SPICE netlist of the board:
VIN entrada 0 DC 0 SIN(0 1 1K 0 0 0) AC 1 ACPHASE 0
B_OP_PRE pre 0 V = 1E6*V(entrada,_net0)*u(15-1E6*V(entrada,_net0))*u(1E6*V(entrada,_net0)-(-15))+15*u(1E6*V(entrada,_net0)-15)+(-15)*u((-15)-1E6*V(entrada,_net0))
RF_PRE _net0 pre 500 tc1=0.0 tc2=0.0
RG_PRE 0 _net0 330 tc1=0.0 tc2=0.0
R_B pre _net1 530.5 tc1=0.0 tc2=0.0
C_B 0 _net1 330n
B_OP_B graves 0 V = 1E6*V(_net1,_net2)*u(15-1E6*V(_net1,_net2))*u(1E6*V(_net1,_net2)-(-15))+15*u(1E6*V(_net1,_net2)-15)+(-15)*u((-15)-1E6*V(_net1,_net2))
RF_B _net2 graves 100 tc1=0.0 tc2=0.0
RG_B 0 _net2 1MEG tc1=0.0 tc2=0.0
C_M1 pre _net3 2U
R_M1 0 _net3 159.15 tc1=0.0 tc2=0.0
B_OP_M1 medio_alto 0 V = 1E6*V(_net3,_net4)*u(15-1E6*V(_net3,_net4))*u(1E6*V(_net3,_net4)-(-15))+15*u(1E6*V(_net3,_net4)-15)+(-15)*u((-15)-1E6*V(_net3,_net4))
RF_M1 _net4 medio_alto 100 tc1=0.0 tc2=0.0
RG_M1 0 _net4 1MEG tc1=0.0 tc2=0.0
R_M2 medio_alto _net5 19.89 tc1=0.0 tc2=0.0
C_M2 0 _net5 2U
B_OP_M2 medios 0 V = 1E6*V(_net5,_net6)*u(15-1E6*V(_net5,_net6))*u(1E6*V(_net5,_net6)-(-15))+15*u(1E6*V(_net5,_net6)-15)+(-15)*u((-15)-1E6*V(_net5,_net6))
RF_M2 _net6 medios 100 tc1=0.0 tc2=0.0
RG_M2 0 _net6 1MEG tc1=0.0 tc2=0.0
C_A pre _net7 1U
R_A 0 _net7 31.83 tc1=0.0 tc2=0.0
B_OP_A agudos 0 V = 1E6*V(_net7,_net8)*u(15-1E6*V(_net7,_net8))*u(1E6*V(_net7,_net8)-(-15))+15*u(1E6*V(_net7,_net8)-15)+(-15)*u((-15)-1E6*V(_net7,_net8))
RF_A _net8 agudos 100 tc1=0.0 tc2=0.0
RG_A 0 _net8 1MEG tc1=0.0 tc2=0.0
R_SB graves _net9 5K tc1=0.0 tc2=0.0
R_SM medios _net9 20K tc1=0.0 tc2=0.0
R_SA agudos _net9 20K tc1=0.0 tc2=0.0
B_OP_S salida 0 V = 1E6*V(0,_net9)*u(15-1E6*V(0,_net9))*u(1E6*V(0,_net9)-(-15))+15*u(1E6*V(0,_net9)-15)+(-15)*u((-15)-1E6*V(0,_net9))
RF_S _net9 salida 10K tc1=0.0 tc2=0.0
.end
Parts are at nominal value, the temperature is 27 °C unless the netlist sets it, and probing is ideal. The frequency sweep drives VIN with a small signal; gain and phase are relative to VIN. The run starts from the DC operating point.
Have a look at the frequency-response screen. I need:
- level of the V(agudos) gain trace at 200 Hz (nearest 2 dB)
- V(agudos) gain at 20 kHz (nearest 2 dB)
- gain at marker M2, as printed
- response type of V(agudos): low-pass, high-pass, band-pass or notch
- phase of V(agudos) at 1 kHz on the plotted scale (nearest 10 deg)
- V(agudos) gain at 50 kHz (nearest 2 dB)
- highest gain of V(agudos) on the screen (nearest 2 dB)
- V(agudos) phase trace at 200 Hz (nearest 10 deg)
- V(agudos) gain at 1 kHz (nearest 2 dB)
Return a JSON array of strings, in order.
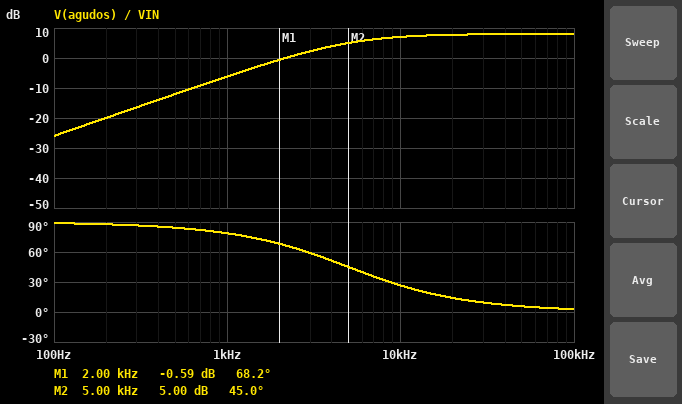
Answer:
["-20 dB", "8 dB", "5.00 dB", "high-pass", "80 deg", "8 dB", "8 dB", "90 deg", "-6 dB"]
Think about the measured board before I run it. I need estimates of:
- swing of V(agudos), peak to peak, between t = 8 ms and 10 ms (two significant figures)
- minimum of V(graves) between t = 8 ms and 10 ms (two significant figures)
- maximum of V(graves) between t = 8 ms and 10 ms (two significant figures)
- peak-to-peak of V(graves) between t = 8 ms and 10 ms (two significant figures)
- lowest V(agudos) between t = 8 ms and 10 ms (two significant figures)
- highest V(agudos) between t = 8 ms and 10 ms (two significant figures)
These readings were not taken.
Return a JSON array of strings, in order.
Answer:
["990 mV", "-1.7 V", "1.7 V", "3.4 V", "-490 mV", "490 mV"]
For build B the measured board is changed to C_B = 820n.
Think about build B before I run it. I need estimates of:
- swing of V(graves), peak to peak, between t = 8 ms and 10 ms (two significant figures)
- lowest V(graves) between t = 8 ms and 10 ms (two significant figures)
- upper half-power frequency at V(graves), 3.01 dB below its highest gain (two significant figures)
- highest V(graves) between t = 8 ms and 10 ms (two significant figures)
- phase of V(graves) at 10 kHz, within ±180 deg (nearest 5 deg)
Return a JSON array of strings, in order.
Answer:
["1.7 V", "-860 mV", "370 Hz", "860 mV", "-90 deg"]
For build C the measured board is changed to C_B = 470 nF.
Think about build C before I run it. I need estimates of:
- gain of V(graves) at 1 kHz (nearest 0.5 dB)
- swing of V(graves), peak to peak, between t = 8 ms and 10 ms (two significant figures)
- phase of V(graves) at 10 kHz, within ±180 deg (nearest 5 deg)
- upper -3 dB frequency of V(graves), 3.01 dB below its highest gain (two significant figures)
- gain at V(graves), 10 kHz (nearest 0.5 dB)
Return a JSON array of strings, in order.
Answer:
["2.5 dB", "2.7 V", "-85 deg", "640 Hz", "-16.0 dB"]
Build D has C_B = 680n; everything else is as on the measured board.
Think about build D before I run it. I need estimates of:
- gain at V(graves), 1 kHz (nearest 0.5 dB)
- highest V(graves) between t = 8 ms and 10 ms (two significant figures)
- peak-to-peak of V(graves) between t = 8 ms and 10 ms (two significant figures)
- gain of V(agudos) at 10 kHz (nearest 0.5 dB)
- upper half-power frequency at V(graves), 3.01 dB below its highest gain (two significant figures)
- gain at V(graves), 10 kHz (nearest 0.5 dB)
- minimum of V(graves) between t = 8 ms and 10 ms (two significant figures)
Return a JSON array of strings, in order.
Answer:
["0 dB", "1.0 V", "2.0 V", "7.0 dB", "440 Hz", "-19.0 dB", "-1.0 V"]
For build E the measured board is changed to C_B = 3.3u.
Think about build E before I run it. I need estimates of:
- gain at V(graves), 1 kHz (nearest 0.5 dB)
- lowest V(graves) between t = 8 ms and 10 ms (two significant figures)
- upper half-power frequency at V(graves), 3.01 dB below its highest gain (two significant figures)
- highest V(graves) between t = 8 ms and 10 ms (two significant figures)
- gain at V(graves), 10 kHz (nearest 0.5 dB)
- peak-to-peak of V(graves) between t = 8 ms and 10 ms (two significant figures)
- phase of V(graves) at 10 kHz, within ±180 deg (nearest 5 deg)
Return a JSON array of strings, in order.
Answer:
["-13.0 dB", "-230 mV", "91 Hz", "230 mV", "-33.0 dB", "460 mV", "-90 deg"]
